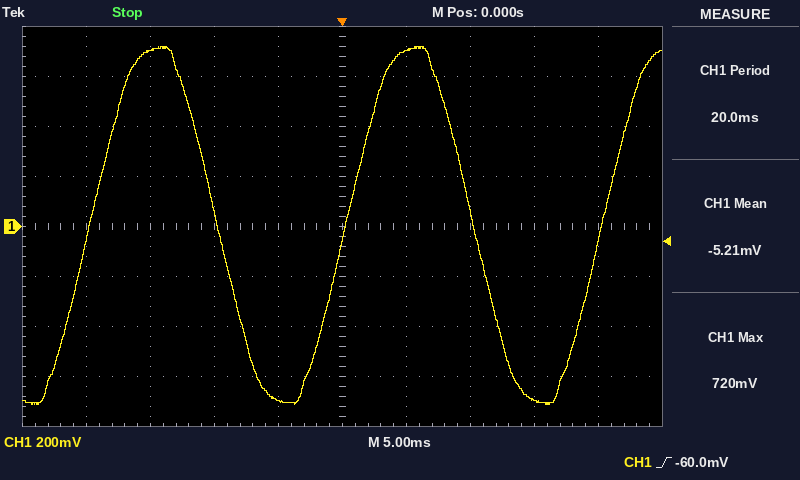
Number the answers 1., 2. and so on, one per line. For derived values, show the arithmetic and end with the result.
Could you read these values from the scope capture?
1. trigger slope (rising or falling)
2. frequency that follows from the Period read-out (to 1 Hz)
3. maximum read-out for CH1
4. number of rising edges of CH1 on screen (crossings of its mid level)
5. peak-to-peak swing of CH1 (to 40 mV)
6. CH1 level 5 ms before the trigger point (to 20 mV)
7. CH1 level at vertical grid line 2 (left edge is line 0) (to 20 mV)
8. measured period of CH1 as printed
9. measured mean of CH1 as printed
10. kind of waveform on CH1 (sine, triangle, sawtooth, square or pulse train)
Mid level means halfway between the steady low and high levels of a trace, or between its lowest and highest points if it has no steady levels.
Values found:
1. rising
2. 1 / 20.0 ms ≈ 50 Hz
3. 720 mV
4. 3
5. 1.44 V
6. -700 mV
7. 700 mV
8. 20.0 ms
9. -5.21 mV
10. sine
